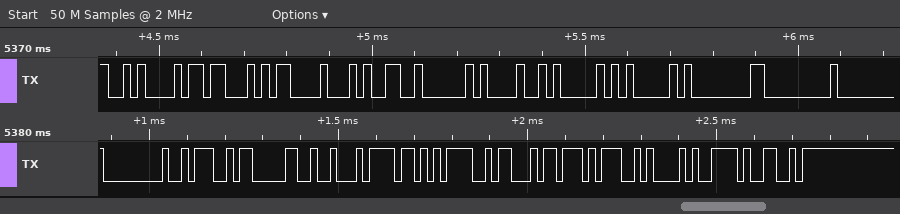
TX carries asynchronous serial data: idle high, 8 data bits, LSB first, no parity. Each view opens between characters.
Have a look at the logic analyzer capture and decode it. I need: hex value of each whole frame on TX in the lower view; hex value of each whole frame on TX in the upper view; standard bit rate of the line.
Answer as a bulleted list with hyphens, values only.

- 00, 3A, 83, 12, 6F, 3D, A3, D7, 0A, 79, A6
- 0A, 1B, 0D, 94, 02, 21, 41, 41, 80, 00
- 57600 baud
